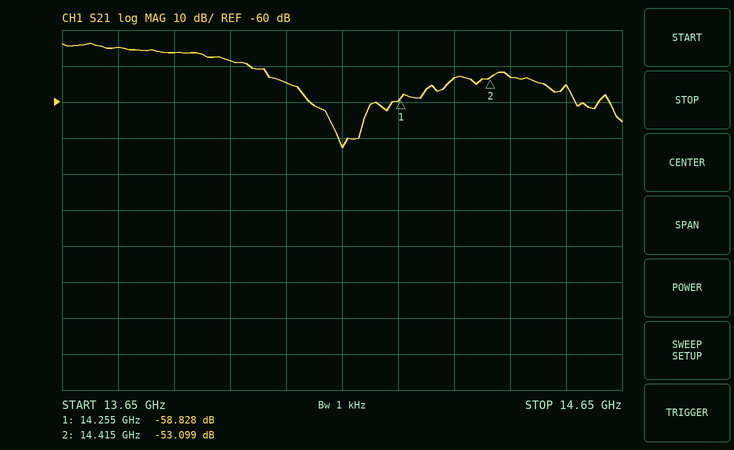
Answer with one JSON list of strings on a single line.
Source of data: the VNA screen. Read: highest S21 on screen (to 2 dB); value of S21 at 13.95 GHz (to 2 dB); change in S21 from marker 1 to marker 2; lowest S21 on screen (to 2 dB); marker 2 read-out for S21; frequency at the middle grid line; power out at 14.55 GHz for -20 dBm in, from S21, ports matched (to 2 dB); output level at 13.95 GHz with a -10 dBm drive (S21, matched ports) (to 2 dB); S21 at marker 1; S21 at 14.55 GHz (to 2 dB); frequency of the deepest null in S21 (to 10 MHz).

["-44 dB", "-48 dB", "5.729 dB", "-72 dB", "-53.099 dB", "14.15 GHz", "-76 dBm", "-58 dBm", "-58.828 dB", "-56 dB", "14.15 GHz"]
